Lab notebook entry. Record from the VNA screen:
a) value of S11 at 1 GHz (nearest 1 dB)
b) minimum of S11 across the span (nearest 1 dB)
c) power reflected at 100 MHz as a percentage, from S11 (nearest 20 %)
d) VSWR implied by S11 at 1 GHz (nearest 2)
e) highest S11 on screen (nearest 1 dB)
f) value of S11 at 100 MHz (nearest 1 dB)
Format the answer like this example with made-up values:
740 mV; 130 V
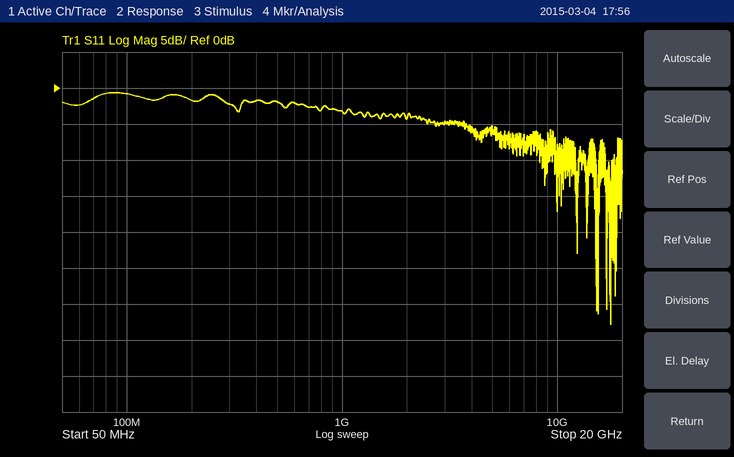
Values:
-3 dB; -33 dB; 80 %; 6; -1 dB; -1 dB
